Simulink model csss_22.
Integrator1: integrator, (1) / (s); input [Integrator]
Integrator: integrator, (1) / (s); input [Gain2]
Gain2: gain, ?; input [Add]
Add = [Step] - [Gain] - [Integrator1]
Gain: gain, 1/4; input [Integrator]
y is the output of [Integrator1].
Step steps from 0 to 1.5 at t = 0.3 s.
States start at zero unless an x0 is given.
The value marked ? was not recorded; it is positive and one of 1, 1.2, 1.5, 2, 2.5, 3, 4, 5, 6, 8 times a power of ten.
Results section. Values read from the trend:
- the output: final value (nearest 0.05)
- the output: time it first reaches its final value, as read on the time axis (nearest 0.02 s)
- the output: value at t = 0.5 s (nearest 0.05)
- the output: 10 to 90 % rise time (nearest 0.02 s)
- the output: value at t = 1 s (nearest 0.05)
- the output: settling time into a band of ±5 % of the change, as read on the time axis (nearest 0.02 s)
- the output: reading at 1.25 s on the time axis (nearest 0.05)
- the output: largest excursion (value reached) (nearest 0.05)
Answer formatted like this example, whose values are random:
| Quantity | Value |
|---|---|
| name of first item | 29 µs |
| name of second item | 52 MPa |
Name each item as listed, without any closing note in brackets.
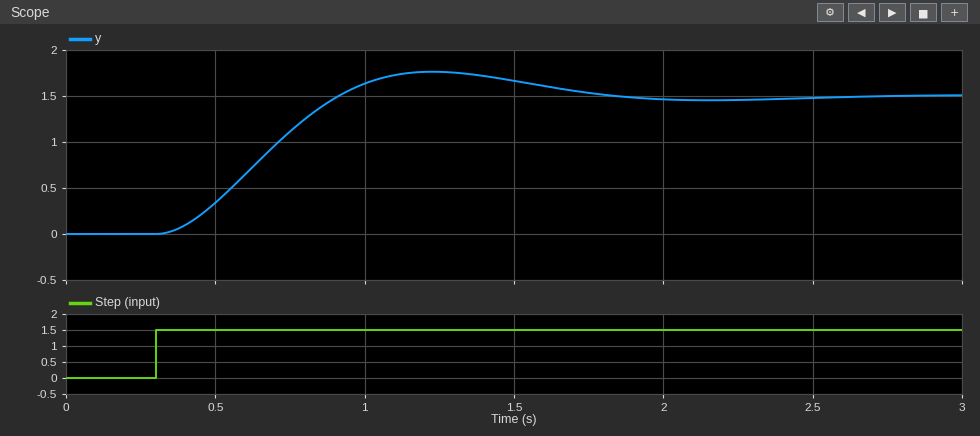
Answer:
| Quantity | Value |
|---|---|
| the output: final value | 1.50 |
| the output: time it first reaches its final value, as read on the time axis | 0.92 s |
| the output: value at t = 0.5 s | 0.35 |
| the output: 10 to 90 % rise time | 0.42 s |
| the output: value at t = 1 s | 1.65 |
| the output: settling time into a band of ±5 % of the change, as read on the time axis | 1.66 s |
| the output: reading at 1.25 s on the time axis | 1.75 |
| the output: largest excursion (value reached) | 1.75 |
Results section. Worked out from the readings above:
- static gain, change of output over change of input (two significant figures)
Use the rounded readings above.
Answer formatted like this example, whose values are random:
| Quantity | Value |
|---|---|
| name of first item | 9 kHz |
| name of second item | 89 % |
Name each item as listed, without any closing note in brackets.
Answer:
| Quantity | Value |
|---|---|
| static gain, change of output over change of input | 1.0 |
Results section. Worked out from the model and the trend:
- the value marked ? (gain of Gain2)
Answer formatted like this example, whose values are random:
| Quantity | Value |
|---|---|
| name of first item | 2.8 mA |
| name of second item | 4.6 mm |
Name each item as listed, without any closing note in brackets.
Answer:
| Quantity | Value |
|---|---|
| the value marked ? | 15 |
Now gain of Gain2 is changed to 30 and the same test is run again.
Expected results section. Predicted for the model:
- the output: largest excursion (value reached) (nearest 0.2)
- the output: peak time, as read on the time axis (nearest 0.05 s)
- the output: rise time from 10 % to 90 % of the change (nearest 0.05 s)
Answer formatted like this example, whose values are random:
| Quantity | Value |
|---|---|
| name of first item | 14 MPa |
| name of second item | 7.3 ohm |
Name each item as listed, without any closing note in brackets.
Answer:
| Quantity | Value |
|---|---|
| the output: largest excursion (value reached) | 1.6 |
| the output: peak time, as read on the time axis | 1.10 s |
| the output: rise time from 10 % to 90 % of the change | 0.40 s |
